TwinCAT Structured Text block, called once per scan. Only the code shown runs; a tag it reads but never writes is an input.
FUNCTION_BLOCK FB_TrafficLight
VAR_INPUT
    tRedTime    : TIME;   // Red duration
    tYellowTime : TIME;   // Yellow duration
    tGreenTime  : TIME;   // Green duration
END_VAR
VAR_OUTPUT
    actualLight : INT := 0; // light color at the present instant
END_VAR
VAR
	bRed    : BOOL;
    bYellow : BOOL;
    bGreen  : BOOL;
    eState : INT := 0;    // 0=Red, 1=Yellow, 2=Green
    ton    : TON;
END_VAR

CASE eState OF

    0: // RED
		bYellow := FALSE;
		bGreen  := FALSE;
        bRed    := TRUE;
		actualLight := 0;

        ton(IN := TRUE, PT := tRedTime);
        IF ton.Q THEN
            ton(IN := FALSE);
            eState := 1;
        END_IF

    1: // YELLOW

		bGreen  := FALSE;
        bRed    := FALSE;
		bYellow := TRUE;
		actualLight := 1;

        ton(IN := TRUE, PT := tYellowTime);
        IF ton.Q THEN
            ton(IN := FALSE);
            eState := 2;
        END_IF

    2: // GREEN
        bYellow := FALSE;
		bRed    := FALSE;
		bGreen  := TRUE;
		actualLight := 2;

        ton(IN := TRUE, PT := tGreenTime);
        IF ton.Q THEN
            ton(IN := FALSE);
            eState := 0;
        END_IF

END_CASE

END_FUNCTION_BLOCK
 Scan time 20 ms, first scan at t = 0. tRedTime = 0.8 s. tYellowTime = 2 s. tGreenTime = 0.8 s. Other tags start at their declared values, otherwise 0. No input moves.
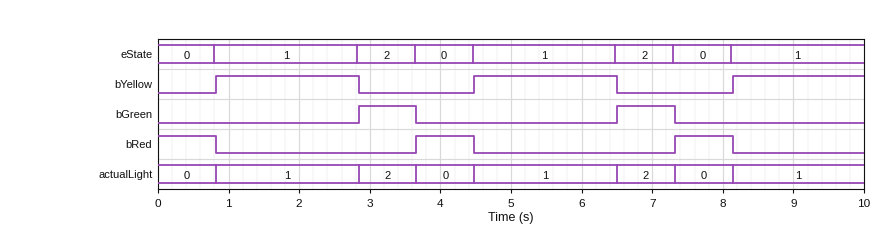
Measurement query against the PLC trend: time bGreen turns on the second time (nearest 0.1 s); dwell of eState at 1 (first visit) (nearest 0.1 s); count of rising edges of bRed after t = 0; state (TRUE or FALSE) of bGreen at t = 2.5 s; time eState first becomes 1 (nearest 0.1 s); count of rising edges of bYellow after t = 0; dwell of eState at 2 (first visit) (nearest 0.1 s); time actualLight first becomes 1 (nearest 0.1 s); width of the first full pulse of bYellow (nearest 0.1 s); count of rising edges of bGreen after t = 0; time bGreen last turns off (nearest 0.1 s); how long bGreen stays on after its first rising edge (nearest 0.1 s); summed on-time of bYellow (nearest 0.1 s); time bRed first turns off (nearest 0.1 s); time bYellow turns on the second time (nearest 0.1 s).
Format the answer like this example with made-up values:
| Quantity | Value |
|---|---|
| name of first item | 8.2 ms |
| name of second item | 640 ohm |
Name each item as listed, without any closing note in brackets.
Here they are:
| Quantity | Value |
|---|---|
| time bGreen turns on the second time | 6.5 s |
| dwell of eState at 1 (first visit) | 2.0 s |
| count of rising edges of bRed after t = 0 | 2 |
| state (TRUE or FALSE) of bGreen at t = 2.5 s | FALSE |
| time eState first becomes 1 | 0.8 s |
| count of rising edges of bYellow after t = 0 | 3 |
| dwell of eState at 2 (first visit) | 0.8 s |
| time actualLight first becomes 1 | 0.8 s |
| width of the first full pulse of bYellow | 2.0 s |
| count of rising edges of bGreen after t = 0 | 2 |
| time bGreen last turns off | 7.3 s |
| how long bGreen stays on after its first rising edge | 0.8 s |
| summed on-time of bYellow | 5.9 s |
| time bRed first turns off | 0.8 s |
| time bYellow turns on the second time | 4.5 s |
